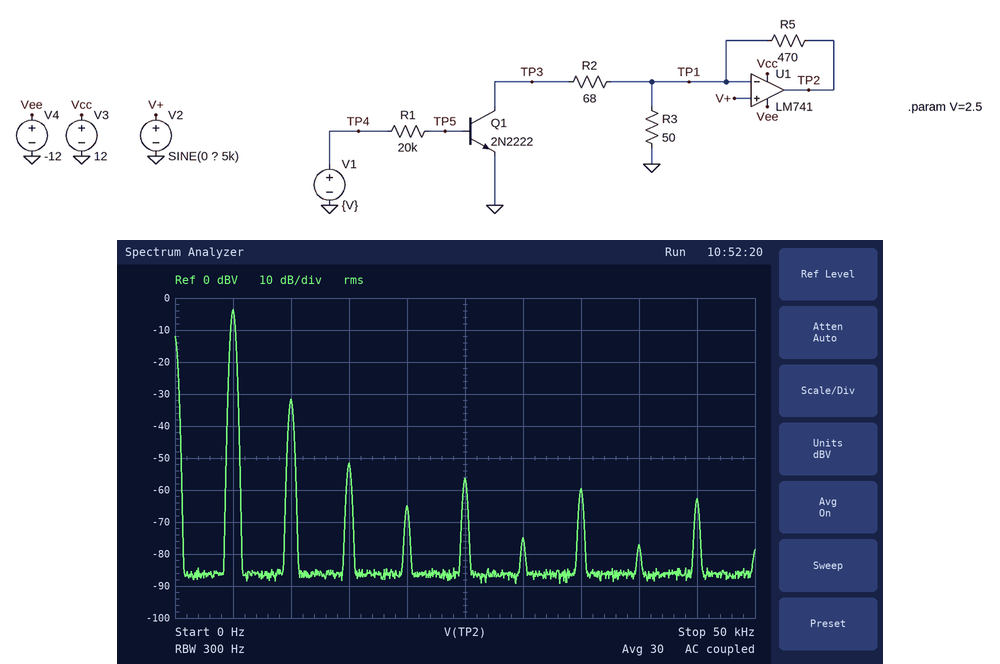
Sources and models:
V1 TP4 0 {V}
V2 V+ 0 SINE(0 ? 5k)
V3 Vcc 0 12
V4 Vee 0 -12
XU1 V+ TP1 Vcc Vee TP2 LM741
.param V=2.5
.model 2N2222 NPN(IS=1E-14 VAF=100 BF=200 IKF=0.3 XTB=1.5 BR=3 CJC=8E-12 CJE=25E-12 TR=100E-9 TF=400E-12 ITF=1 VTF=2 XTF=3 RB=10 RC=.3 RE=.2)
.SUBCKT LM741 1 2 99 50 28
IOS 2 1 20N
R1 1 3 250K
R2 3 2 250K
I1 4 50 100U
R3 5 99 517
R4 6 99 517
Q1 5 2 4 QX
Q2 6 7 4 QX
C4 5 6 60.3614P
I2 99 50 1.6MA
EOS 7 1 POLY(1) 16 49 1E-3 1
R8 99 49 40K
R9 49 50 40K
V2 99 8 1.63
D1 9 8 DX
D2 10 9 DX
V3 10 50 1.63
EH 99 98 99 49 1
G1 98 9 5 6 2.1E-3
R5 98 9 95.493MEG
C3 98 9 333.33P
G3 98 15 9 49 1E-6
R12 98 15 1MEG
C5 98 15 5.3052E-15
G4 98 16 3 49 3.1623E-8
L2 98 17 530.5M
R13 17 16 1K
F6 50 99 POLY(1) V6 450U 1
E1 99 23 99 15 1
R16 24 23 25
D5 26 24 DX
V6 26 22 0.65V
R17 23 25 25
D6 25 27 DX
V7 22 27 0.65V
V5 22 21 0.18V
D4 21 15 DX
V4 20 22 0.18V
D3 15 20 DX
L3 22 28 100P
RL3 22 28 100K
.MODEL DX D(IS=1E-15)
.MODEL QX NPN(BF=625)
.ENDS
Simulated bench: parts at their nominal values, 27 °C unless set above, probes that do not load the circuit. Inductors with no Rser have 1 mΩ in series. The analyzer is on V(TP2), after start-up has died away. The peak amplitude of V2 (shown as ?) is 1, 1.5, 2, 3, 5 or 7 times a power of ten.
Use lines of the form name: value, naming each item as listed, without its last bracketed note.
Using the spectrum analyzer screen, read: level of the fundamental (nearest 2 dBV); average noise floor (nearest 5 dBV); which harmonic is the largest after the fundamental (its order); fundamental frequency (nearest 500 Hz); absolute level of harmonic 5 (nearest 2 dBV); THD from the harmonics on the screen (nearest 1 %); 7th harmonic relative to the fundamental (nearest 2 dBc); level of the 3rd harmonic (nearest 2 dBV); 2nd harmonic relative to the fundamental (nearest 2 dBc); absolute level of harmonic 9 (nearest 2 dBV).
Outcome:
level of the fundamental: -4 dBV
average noise floor: -85 dBV
which harmonic is the largest after the fundamental: 2
fundamental frequency: 5.0 kHz
absolute level of harmonic 5: -56 dBV
THD from the harmonics on the screen: 4 %
7th harmonic relative to the fundamental: -56 dBc
level of the 3rd harmonic: -52 dBV
2nd harmonic relative to the fundamental: -28 dBc
absolute level of harmonic 9: -62 dBV
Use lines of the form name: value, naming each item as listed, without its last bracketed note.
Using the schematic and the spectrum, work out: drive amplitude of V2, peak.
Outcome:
drive amplitude of V2, peak: 70 mV
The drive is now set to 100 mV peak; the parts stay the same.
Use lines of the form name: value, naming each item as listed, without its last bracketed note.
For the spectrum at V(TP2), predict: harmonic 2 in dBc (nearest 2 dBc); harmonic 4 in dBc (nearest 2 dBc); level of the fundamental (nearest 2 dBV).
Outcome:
harmonic 2 in dBc: -26 dBc
harmonic 4 in dBc: -54 dBc
level of the fundamental: 0 dBV
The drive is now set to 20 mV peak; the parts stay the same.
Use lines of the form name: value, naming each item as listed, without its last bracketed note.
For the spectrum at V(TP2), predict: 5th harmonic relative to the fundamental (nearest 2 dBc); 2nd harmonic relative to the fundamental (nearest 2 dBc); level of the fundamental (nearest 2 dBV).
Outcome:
5th harmonic relative to the fundamental: -56 dBc
2nd harmonic relative to the fundamental: -38 dBc
level of the fundamental: -14 dBV
